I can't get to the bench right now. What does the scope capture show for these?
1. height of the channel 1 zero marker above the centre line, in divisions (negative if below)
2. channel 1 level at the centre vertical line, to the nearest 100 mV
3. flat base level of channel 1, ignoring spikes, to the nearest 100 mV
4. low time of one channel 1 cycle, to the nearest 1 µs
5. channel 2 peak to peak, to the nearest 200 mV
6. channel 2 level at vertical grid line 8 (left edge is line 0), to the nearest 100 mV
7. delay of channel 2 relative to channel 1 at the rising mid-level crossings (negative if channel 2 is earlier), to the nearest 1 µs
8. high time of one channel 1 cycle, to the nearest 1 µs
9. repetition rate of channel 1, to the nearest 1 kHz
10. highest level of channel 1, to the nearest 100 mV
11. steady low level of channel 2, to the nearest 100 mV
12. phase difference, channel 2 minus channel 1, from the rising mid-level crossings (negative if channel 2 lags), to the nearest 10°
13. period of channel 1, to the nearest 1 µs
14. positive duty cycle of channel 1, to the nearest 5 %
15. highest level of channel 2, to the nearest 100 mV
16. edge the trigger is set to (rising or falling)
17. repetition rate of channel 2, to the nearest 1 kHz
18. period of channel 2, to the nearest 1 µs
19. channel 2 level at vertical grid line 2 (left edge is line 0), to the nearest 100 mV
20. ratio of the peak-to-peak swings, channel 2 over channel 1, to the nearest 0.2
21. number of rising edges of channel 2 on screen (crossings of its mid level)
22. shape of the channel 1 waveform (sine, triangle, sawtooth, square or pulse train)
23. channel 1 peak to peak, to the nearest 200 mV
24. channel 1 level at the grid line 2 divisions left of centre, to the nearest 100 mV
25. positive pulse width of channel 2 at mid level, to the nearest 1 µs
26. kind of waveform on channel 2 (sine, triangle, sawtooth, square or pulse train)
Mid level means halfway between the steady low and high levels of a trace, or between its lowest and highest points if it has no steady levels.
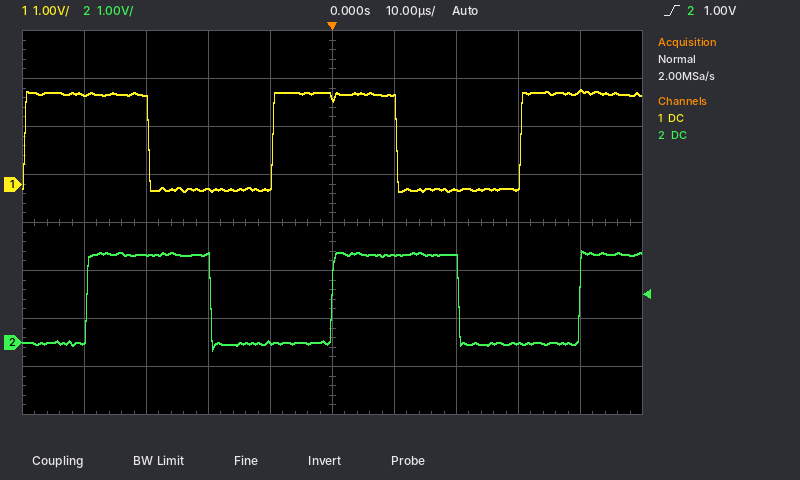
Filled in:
+0.8 div
1.8 V
-100 mV
20 µs
2.0 V
0.0 V
+10 µs
20 µs
25 kHz
2.0 V
0.0 V
-90°
40 µs
50 %
1.9 V
rising
25 kHz
40 µs
1.8 V
1.0
3
square
2.2 V
-100 mV
20 µs
square
